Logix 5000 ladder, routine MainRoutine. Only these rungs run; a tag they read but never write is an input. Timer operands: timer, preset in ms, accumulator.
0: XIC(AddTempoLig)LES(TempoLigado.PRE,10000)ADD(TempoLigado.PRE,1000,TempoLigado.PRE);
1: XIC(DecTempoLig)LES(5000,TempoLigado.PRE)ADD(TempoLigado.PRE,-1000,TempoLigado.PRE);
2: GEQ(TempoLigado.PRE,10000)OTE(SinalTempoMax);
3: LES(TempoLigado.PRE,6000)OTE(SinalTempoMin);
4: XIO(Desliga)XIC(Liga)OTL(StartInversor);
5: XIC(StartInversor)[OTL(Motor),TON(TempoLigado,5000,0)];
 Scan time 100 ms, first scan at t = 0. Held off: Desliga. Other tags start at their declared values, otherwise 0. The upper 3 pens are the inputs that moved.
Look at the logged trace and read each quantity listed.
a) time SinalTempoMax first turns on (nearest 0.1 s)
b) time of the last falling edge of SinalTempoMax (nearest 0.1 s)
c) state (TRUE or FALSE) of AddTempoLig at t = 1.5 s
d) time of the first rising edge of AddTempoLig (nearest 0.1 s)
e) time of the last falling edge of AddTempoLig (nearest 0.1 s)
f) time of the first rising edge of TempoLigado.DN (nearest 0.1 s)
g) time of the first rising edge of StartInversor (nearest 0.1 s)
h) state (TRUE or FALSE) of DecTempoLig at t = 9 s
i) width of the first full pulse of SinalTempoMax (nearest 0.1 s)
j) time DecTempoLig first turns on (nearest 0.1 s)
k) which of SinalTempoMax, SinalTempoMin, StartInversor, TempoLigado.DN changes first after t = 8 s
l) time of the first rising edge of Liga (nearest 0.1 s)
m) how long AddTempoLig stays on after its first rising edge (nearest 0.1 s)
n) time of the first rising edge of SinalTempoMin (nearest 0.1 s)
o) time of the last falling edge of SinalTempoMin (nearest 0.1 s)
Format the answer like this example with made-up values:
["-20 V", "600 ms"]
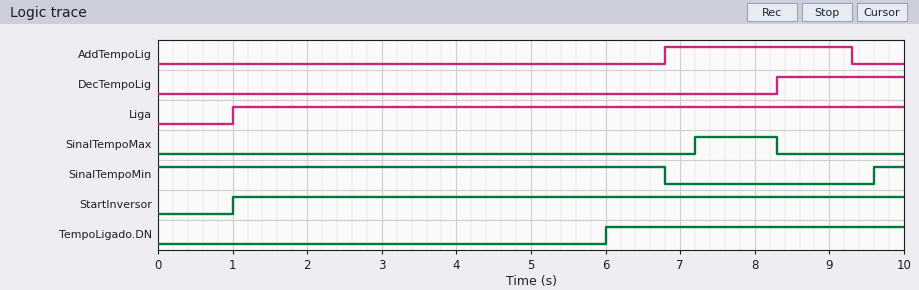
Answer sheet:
["7.2 s", "8.3 s", "FALSE", "6.8 s", "9.3 s", "6.0 s", "1.0 s", "TRUE", "1.1 s", "8.3 s", "SinalTempoMax", "1.0 s", "2.5 s", "9.6 s", "6.8 s"]
